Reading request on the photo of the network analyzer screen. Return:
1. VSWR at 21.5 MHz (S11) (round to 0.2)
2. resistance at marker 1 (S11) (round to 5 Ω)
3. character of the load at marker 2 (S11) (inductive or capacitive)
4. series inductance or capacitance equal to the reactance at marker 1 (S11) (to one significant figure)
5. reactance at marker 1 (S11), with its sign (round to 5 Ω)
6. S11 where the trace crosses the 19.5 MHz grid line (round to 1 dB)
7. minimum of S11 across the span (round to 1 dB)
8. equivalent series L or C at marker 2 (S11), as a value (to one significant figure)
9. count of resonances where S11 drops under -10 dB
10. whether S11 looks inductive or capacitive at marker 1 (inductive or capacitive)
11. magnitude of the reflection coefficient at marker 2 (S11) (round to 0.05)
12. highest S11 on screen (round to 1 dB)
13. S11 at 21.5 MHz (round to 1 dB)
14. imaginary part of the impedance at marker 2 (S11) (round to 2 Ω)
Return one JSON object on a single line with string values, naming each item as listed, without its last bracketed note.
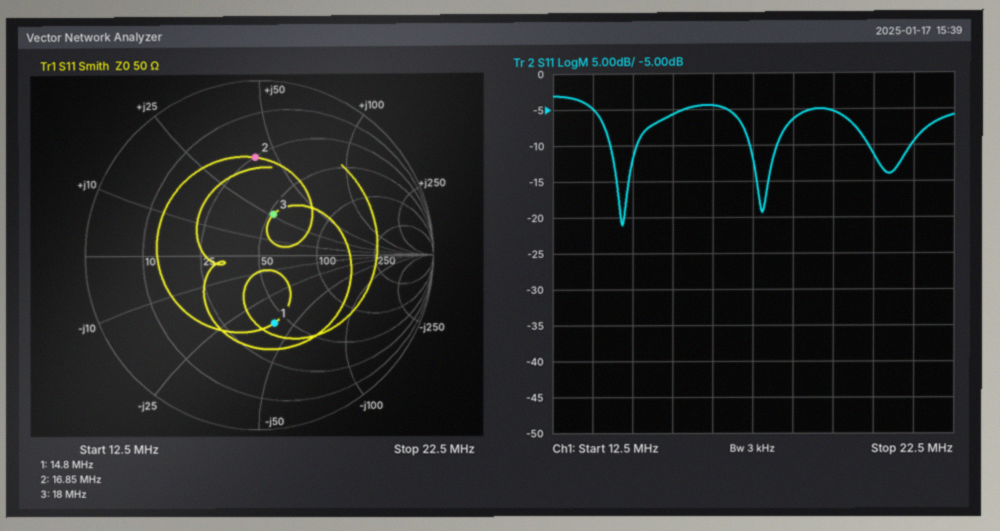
{"VSWR at 21.5 MHz (S11)": "2.0", "resistance at marker 1 (S11)": "45 Ω", "character of the load at marker 2 (S11)": "inductive", "series inductance or capacitance equal to the reactance at marker 1 (S11)": "300 pF", "reactance at marker 1 (S11), with its sign": "-40 Ω", "S11 where the trace crosses the 19.5 MHz grid line": "-5 dB", "minimum of S11 across the span": "-21 dB", "equivalent series L or C at marker 2 (S11), as a value": "400 nH", "count of resonances where S11 drops under -10 dB": "3", "whether S11 looks inductive or capacitive at marker 1": "capacitive", "magnitude of the reflection coefficient at marker 2 (S11)": "0.55", "highest S11 on screen": "-3 dB", "S11 at 21.5 MHz": "-10 dB", "imaginary part of the impedance at marker 2 (S11)": "+42 Ω"}
